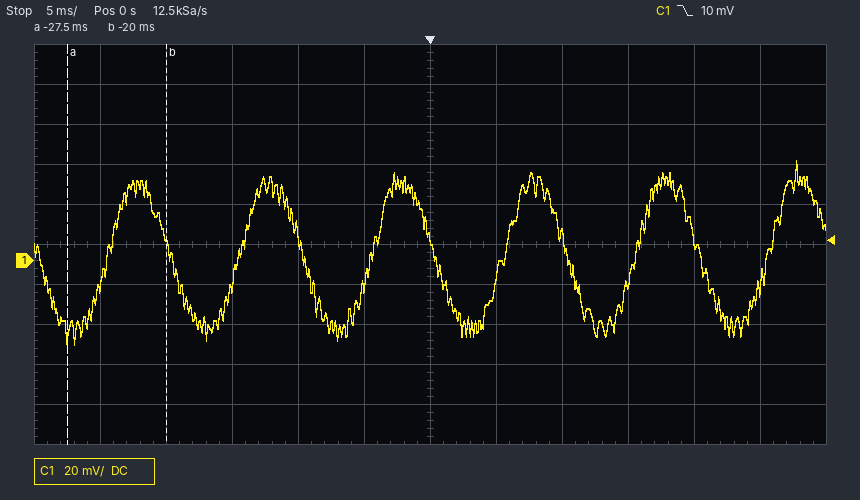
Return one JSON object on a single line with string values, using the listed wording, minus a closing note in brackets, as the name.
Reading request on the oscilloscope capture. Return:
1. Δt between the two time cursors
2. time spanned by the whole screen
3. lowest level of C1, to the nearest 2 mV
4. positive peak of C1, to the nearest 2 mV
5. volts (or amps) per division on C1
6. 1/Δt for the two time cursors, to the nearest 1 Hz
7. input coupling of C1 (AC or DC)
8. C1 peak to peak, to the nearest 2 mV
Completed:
{"Δt between the two time cursors": "7.5 ms", "time spanned by the whole screen": "60 ms", "lowest level of C1, to the nearest 2 mV": "-42 mV", "positive peak of C1, to the nearest 2 mV": "50 mV", "volts (or amps) per division on C1": "20 mV", "1/Δt for the two time cursors, to the nearest 1 Hz": "133 Hz", "input coupling of C1": "DC", "C1 peak to peak, to the nearest 2 mV": "92 mV"}
